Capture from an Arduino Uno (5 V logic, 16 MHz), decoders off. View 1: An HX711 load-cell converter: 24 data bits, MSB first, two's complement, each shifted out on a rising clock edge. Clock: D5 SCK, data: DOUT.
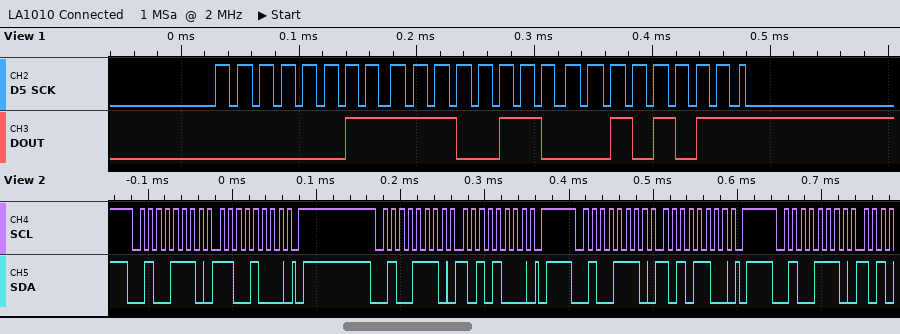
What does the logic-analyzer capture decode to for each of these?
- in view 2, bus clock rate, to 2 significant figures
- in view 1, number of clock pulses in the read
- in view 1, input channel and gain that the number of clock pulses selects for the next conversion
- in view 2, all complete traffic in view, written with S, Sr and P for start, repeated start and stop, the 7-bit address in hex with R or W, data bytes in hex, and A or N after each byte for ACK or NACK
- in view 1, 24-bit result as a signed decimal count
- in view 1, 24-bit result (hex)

100 kHz
25
channel A, gain 128
S 27W A C8 A P S 27W A A8 A P S 27W A AC A P S 27W A
255531
0x03E62B
